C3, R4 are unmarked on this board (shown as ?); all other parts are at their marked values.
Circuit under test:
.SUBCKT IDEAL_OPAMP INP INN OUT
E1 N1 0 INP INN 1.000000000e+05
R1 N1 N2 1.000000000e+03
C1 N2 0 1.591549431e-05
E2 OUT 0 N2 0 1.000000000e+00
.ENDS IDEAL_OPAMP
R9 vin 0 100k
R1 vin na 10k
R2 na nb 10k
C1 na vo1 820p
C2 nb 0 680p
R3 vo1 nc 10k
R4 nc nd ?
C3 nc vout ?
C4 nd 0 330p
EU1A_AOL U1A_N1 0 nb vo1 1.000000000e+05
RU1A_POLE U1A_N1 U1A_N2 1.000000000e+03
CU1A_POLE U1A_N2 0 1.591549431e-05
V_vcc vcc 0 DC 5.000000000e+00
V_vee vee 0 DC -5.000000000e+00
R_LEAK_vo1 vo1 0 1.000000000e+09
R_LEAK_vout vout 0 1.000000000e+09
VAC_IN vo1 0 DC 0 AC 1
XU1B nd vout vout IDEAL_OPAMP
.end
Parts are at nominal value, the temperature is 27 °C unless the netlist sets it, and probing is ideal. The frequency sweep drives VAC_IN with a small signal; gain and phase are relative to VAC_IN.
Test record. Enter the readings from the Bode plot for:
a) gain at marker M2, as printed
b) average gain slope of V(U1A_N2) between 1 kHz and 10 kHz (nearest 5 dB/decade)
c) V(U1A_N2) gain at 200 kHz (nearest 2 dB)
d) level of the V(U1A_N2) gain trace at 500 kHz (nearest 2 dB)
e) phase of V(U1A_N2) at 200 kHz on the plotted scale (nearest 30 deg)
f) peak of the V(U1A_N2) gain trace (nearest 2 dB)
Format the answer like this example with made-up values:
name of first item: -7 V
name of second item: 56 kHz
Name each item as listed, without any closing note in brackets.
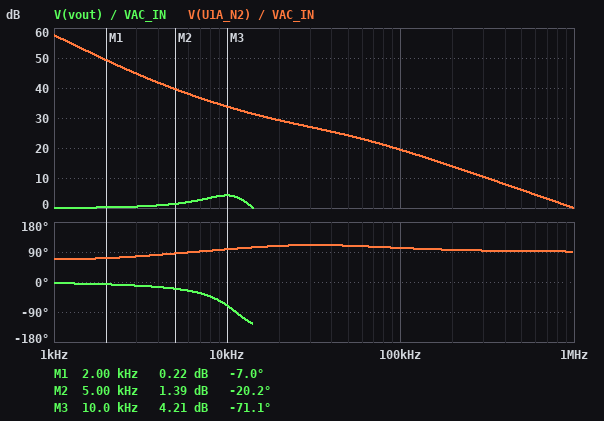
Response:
gain at marker M2, as printed: 1.39 dB
average gain slope of V(U1A_N2) between 1 kHz and 10 kHz: -25 dB/decade
V(U1A_N2) gain at 200 kHz: 14 dB
level of the V(U1A_N2) gain trace at 500 kHz: 6 dB
phase of V(U1A_N2) at 200 kHz on the plotted scale: 90 deg
peak of the V(U1A_N2) gain trace: 58 dB
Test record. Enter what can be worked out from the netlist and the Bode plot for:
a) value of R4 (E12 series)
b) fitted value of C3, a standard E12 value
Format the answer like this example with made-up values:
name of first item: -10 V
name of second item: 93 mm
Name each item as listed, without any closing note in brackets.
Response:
value of R4: 18 kΩ
fitted value of C3, a standard E12 value: 3.3 nF
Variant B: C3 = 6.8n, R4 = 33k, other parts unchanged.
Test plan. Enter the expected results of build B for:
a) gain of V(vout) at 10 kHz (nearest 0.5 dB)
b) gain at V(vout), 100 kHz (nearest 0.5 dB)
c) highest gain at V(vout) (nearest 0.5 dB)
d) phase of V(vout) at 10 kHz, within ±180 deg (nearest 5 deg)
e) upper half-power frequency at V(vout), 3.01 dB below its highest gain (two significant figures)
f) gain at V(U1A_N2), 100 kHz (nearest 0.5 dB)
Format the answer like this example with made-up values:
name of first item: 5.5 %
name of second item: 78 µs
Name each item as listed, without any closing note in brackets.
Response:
gain of V(vout) at 10 kHz: -6.5 dB
gain at V(vout), 100 kHz: -49.5 dB
highest gain at V(vout): 6.0 dB
phase of V(vout) at 10 kHz, within ±180 deg: -155 deg
upper half-power frequency at V(vout), 3.01 dB below its highest gain: 6.8 kHz
gain at V(U1A_N2), 100 kHz: 19.5 dB
